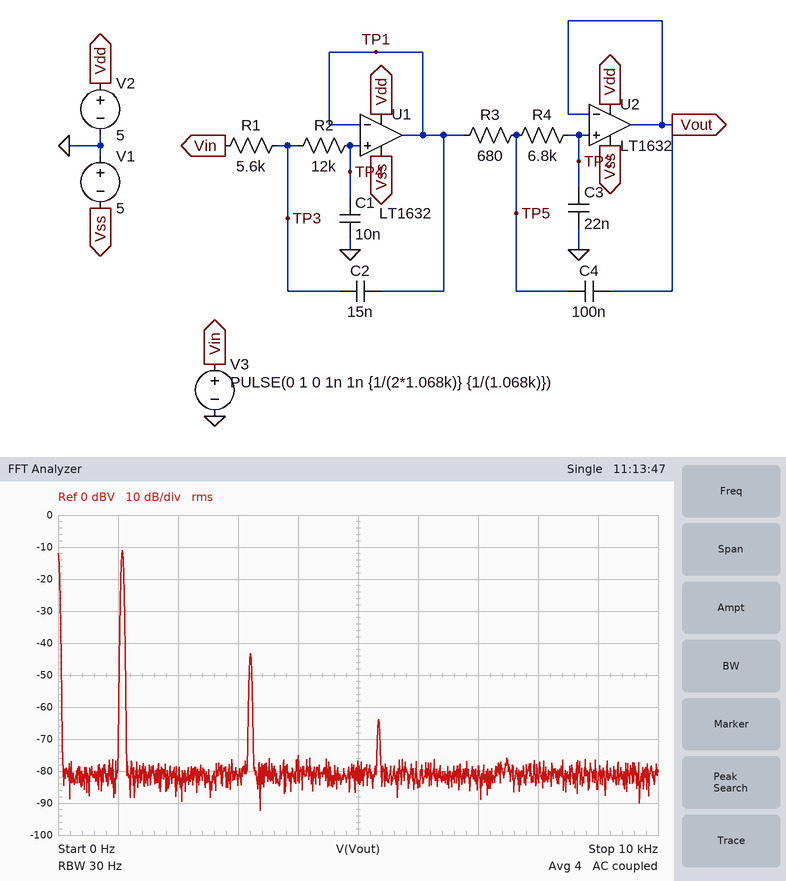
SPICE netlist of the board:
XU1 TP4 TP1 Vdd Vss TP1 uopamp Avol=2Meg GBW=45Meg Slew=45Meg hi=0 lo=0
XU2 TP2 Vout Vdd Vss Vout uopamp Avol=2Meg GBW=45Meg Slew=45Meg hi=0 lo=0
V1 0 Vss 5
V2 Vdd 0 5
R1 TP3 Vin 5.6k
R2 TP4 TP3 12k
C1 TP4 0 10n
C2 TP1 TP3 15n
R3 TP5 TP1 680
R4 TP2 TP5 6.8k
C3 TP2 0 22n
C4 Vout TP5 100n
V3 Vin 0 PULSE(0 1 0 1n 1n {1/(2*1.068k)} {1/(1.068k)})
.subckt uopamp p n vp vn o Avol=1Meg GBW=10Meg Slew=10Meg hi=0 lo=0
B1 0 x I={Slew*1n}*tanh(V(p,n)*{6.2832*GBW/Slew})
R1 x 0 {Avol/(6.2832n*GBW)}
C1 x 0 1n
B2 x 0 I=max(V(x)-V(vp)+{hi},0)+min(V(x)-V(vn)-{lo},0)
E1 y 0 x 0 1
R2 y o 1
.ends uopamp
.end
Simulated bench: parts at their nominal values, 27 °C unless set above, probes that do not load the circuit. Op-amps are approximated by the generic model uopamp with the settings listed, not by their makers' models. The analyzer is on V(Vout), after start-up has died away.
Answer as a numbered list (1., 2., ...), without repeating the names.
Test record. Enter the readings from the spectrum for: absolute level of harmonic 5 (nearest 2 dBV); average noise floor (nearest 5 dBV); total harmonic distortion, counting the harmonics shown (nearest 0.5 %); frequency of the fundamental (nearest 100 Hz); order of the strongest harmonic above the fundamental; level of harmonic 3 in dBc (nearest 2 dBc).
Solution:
1. -64 dBV
2. -80 dBV
3. 2.5 %
4. 1.1 kHz
5. 3
6. -32 dBc
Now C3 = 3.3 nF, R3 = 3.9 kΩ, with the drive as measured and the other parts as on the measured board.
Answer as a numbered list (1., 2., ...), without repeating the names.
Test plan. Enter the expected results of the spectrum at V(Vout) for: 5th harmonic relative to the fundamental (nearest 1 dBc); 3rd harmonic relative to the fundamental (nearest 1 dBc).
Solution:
1. -56 dBc
2. -33 dBc
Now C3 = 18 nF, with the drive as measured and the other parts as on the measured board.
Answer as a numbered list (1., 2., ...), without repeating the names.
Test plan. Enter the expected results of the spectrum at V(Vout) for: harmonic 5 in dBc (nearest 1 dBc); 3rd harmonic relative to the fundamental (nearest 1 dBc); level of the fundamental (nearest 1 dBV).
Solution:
1. -52 dBc
2. -31 dBc
3. -10 dBV
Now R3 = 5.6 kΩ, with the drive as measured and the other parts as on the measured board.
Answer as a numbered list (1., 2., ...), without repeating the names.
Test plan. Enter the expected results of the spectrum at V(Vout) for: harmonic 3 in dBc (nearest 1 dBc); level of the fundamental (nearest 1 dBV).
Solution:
1. -41 dBc
2. -20 dBV
